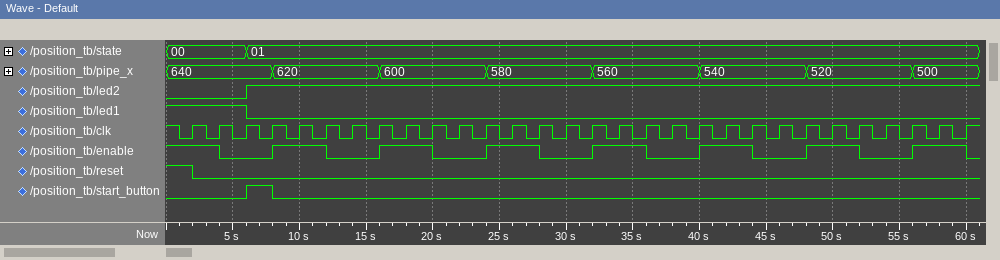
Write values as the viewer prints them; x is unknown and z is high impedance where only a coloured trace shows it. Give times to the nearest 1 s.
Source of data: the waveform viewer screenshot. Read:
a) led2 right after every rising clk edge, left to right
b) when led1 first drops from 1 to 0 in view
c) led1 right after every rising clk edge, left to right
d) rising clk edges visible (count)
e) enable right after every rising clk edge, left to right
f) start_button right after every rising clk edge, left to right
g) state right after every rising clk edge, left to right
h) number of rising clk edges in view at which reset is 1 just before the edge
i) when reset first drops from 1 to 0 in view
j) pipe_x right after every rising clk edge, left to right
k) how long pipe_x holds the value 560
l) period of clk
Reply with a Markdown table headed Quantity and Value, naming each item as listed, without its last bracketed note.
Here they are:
| Quantity | Value |
|---|---|
| led2 right after every rising clk edge, left to right | 0 0 1 1 1 1 1 1 1 1 1 1 1 1 1 1 1 1 1 1 1 1 1 1 1 1 1 1 1 1 |
| when led1 first drops from 1 to 0 in view | 6 s |
| led1 right after every rising clk edge, left to right | 1 1 0 0 0 0 0 0 0 0 0 0 0 0 0 0 0 0 0 0 0 0 0 0 0 0 0 0 0 0 |
| rising clk edges visible | 30 |
| enable right after every rising clk edge, left to right | 1 0 0 1 1 0 0 1 1 0 0 1 1 0 0 1 1 0 0 1 1 0 0 1 1 0 0 1 1 0 |
| start_button right after every rising clk edge, left to right | 0 0 1 0 0 0 0 0 0 0 0 0 0 0 0 0 0 0 0 0 0 0 0 0 0 0 0 0 0 0 |
| state right after every rising clk edge, left to right | 00, 00, 01, 01, 01, 01, 01, 01, 01, 01, 01, 01, 01, 01, 01, 01, 01, 01, 01, 01, 01, 01, 01, 01, 01, 01, 01, 01, 01, 01 |
| number of rising clk edges in view at which reset is 1 just before the edge | 1 |
| when reset first drops from 1 to 0 in view | 2 s |
| pipe_x right after every rising clk edge, left to right | 640, 640, 640, 620, 620, 620, 620, 600, 600, 600, 600, 580, 580, 580, 580, 560, 560, 560, 560, 540, 540, 540, 540, 520, 520, 520, 520, 500, 500, 500 |
| how long pipe_x holds the value 560 | 8 s |
| period of clk | 2 s |
